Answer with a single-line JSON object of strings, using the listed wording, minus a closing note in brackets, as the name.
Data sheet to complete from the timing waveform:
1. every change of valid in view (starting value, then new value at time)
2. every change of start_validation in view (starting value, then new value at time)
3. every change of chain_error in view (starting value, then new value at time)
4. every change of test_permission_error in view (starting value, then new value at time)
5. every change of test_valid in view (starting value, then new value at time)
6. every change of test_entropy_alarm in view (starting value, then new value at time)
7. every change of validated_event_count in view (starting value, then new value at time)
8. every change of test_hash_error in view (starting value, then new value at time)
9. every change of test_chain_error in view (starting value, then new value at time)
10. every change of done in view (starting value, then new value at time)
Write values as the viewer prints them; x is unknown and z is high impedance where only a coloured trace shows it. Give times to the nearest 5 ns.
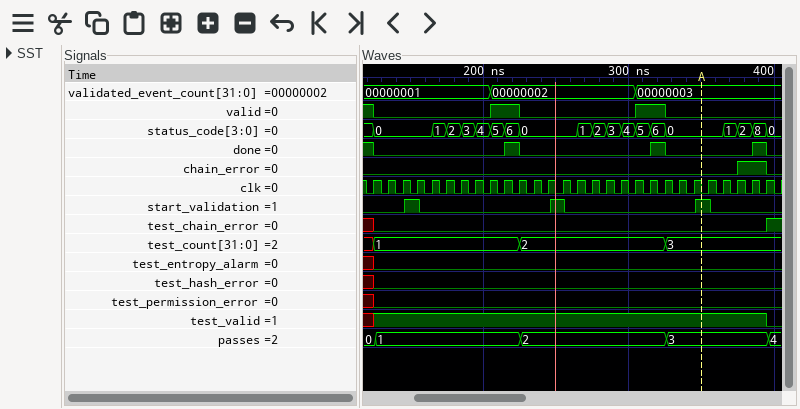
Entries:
{"every change of valid in view": "1, 0 at 125 ns, 1 at 205 ns, 0 at 225 ns, 1 at 305 ns, 0 at 325 ns", "every change of start_validation in view": "0, 1 at 145 ns, 0 at 155 ns, 1 at 245 ns, 0 at 255 ns, 1 at 345 ns, 0 at 355 ns", "every change of chain_error in view": "0, 1 at 375 ns, 0 at 395 ns", "every change of test_permission_error in view": "x, 0 at 125 ns", "every change of test_valid in view": "x, 1 at 125 ns, 0 at 395 ns", "every change of test_entropy_alarm in view": "x, 0 at 125 ns", "every change of validated_event_count in view": "00000001, 00000002 at 205 ns, 00000003 at 305 ns", "every change of test_hash_error in view": "x, 0 at 125 ns", "every change of test_chain_error in view": "x, 0 at 125 ns, 1 at 395 ns", "every change of done in view": "1, 0 at 125 ns, 1 at 215 ns, 0 at 225 ns, 1 at 315 ns, 0 at 325 ns, 1 at 385 ns, 0 at 395 ns"}
